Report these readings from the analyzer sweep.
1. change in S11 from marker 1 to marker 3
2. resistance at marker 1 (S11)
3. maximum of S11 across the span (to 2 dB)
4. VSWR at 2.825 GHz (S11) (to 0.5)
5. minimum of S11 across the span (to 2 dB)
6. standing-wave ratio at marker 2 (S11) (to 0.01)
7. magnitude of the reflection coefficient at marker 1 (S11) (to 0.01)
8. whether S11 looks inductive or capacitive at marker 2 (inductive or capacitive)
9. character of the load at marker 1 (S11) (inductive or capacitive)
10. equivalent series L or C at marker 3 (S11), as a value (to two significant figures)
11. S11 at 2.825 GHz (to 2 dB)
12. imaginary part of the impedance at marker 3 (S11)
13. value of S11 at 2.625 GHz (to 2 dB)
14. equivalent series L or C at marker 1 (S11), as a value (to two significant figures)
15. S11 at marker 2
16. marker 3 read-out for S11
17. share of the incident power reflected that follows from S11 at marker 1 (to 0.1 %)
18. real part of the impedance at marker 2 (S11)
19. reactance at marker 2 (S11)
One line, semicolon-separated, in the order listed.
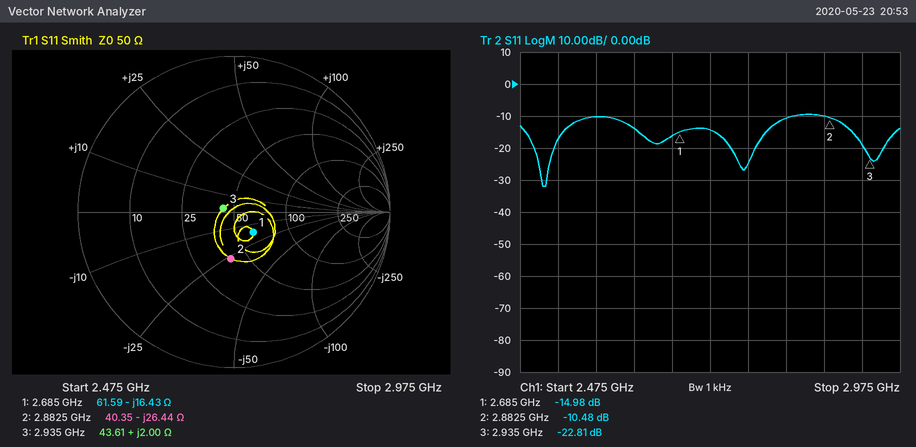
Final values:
-7.83 dB; 61.59 Ω; -10 dB; 2.0; -32 dB; 1.85; 0.18; capacitive; capacitive; 110 pH; -10 dB; +2.00 Ω; -14 dB; 3.6 pF; -10.48 dB; -22.81 dB; 3.2 %; 40.35 Ω; -26.44 Ω
